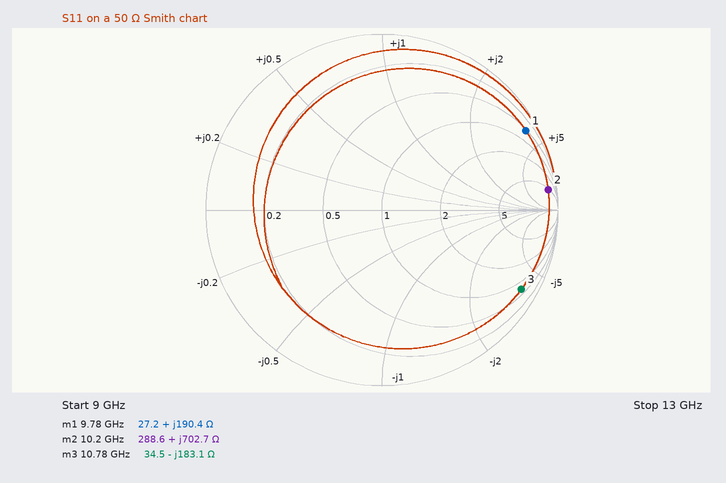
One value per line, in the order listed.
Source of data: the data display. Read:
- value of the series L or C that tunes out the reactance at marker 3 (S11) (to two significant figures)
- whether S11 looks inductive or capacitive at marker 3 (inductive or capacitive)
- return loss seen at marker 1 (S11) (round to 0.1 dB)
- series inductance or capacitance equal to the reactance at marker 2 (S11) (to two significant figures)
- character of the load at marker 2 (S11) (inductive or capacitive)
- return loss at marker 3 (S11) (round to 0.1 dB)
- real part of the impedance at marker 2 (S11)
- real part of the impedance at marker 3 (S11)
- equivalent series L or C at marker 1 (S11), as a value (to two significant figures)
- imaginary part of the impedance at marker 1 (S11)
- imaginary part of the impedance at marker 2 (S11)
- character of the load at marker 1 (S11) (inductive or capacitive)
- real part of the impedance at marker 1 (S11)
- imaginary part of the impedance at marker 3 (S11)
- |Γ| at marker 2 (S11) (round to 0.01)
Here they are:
2.7 nH
capacitive
0.6 dB
11 nH
inductive
0.8 dB
288.6 Ω
34.5 Ω
3.1 nH
+190.4 Ω
+702.7 Ω
inductive
27.2 Ω
-183.1 Ω
0.95
